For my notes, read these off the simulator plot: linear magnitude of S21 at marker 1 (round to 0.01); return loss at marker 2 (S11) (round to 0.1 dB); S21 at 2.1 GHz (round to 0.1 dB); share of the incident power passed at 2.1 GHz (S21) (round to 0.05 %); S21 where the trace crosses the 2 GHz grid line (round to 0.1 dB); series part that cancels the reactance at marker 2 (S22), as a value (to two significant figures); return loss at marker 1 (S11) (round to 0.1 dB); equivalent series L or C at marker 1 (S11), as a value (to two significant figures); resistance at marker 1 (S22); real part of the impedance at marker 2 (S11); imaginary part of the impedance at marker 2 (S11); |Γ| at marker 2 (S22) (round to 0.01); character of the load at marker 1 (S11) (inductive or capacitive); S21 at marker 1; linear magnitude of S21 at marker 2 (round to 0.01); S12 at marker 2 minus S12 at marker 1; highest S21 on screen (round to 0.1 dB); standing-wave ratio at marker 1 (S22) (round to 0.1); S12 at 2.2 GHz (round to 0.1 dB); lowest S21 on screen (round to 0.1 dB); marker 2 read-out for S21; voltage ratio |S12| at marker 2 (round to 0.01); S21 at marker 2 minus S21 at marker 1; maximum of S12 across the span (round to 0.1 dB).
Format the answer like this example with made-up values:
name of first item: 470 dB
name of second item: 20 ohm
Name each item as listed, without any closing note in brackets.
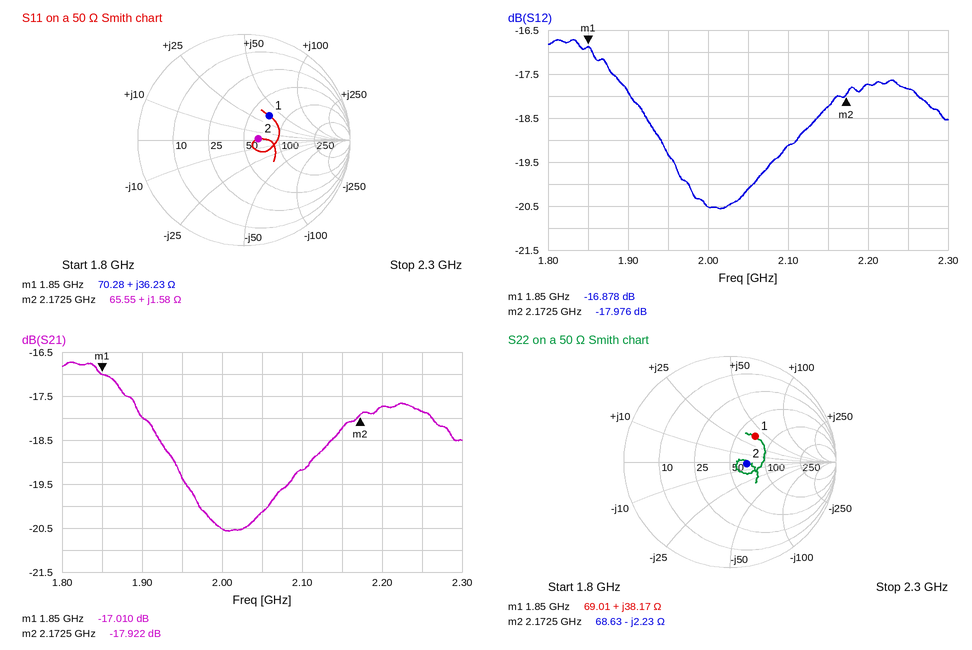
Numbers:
linear magnitude of S21 at marker 1: 0.14
return loss at marker 2 (S11): 17.4 dB
S21 at 2.1 GHz: -19.2 dB
share of the incident power passed at 2.1 GHz (S21): 1.20 %
S21 where the trace crosses the 2 GHz grid line: -20.5 dB
series part that cancels the reactance at marker 2 (S22), as a value: 160 pH
return loss at marker 1 (S11): 9.6 dB
equivalent series L or C at marker 1 (S11), as a value: 3.1 nH
resistance at marker 1: 69.01 Ω
real part of the impedance at marker 2: 65.55 Ω
imaginary part of the impedance at marker 2: +1.58 Ω
|Γ| at marker 2 (S22): 0.16
character of the load at marker 1 (S11): inductive
S21 at marker 1: -17.010 dB
linear magnitude of S21 at marker 2: 0.13
S12 at marker 2 minus S12 at marker 1: -1.098 dB
highest S21 on screen: -16.7 dB
standing-wave ratio at marker 1 (S22): 2.0
S12 at 2.2 GHz: -17.7 dB
lowest S21 on screen: -20.6 dB
marker 2 read-out for S21: -17.922 dB
voltage ratio |S12| at marker 2: 0.13
S21 at marker 2 minus S21 at marker 1: -0.912 dB
maximum of S12 across the span: -16.7 dB
